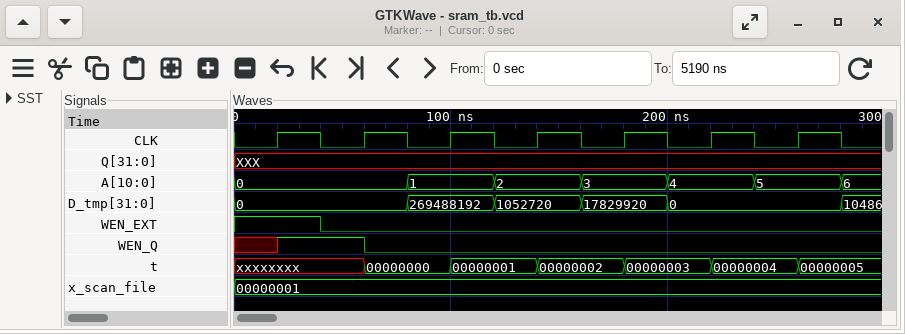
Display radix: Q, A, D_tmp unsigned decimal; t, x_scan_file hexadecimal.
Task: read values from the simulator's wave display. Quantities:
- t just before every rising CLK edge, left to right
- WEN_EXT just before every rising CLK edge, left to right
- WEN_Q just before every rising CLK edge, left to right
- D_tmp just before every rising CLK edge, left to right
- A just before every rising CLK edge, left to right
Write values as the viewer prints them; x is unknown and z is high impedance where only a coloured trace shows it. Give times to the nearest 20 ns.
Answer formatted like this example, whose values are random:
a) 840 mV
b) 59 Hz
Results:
a) xxxxxxxx, xxxxxxxx, 00000000, 00000001, 00000002, 00000003, 00000004
b) 1 0 0 0 0 0 0
c) x 1 0 0 0 0 0
d) 0, 0, 269488192, 1052720, 17829920, 0, 0
e) 0, 0, 1, 2, 3, 4, 5
